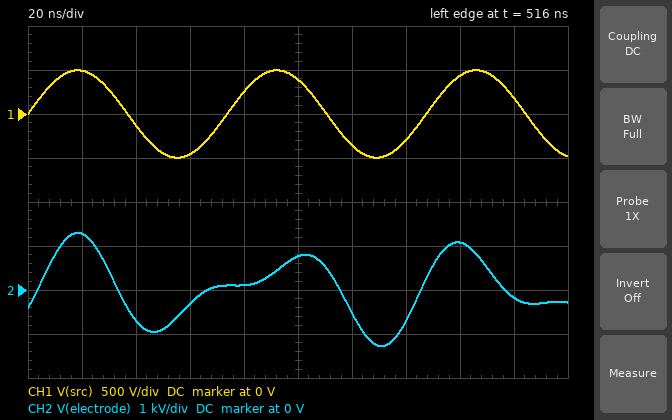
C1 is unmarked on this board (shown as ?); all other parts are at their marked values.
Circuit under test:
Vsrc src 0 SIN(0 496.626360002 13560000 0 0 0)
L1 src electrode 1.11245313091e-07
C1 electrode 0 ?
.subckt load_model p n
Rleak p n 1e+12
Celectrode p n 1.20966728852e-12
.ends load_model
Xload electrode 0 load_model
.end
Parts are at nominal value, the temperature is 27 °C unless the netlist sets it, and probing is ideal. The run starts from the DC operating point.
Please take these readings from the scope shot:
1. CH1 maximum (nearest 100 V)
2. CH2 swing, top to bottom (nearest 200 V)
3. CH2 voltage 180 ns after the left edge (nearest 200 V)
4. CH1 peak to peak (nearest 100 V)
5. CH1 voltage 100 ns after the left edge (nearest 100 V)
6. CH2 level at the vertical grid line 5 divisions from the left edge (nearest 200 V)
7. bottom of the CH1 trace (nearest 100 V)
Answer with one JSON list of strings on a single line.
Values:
["500 V", "2.6 kV", "-200 V", "1.0 kV", "400 V", "800 V", "-500 V"]
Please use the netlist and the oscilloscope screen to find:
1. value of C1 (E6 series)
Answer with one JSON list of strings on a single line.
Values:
["470 pF"]
